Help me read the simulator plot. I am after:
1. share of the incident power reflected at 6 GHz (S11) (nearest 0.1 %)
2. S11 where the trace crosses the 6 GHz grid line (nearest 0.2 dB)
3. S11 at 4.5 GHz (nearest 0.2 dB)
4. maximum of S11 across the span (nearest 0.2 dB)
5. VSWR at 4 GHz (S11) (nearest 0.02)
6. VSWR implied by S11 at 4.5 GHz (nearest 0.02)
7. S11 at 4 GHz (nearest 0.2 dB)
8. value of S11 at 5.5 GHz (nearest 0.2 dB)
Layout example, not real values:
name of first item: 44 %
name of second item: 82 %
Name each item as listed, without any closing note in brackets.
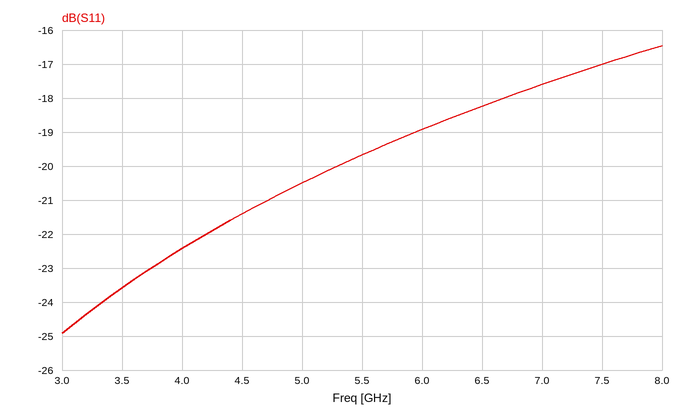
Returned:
share of the incident power reflected at 6 GHz (S11): 1.3 %
S11 where the trace crosses the 6 GHz grid line: -19.0 dB
S11 at 4.5 GHz: -21.4 dB
maximum of S11 across the span: -16.4 dB
VSWR at 4 GHz (S11): 1.16
VSWR implied by S11 at 4.5 GHz: 1.18
S11 at 4 GHz: -22.4 dB
value of S11 at 5.5 GHz: -19.6 dB
